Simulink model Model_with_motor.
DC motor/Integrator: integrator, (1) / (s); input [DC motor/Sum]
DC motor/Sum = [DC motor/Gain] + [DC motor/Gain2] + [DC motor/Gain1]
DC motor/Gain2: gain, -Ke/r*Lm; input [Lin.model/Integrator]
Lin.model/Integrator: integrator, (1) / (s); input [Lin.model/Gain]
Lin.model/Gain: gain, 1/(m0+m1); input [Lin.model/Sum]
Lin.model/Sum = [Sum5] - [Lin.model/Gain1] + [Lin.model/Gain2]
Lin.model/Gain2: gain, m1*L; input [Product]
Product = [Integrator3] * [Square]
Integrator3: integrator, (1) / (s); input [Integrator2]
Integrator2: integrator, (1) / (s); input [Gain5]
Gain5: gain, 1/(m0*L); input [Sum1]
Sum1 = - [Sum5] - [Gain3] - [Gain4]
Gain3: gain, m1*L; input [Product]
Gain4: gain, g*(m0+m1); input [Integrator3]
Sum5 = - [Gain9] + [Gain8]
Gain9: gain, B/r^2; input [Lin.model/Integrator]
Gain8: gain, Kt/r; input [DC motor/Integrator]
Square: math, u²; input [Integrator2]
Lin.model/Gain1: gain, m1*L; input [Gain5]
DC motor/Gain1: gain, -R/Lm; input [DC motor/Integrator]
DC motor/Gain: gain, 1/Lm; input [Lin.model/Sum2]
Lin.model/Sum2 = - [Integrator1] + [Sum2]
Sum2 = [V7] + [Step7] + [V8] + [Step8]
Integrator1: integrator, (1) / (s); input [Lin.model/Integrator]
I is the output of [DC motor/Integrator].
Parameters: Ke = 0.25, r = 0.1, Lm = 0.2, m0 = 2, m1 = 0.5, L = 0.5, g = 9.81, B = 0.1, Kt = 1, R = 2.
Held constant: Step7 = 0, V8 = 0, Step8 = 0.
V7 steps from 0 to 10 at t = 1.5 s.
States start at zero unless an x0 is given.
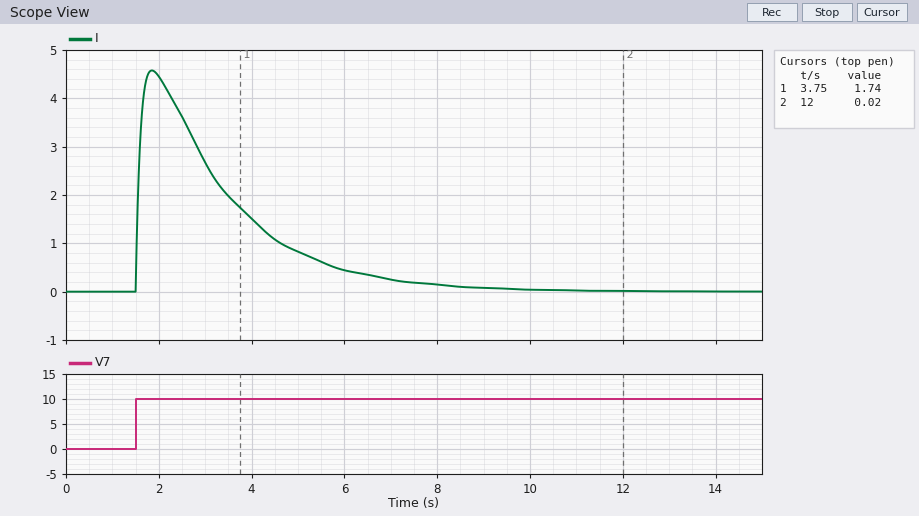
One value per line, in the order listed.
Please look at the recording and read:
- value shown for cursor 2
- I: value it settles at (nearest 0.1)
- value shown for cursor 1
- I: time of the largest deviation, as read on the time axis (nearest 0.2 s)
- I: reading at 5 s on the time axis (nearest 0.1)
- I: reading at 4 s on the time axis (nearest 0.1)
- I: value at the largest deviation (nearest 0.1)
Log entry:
0.02
0.0
1.74
1.8 s
0.8
1.5
4.6
